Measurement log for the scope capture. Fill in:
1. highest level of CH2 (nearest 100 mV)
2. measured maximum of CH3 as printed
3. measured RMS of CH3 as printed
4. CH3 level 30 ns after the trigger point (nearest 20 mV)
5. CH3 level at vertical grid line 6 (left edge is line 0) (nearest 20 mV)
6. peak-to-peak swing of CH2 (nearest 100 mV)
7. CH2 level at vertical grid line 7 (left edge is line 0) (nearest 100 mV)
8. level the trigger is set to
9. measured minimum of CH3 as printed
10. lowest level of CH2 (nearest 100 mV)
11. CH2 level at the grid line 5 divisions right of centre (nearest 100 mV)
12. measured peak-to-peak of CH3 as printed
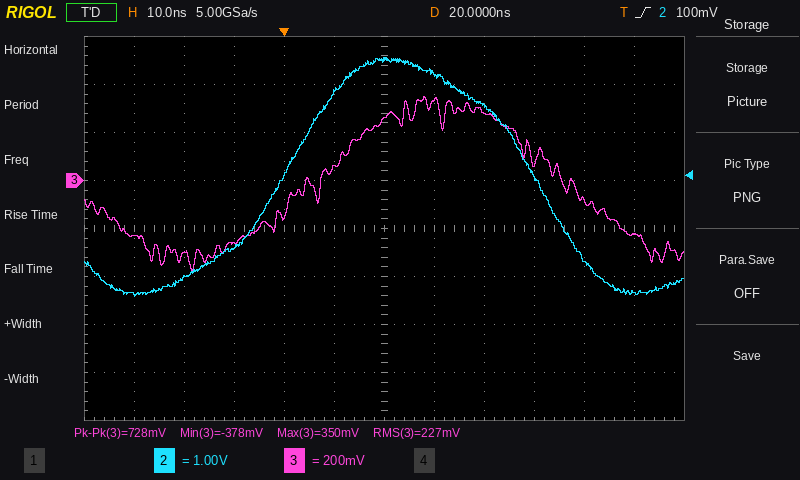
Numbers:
2.6 V
350 mV
227 mV
340 mV
260 mV
5.0 V
2.2 V
100 mV
-378 mV
-2.4 V
-2.3 V
728 mV
